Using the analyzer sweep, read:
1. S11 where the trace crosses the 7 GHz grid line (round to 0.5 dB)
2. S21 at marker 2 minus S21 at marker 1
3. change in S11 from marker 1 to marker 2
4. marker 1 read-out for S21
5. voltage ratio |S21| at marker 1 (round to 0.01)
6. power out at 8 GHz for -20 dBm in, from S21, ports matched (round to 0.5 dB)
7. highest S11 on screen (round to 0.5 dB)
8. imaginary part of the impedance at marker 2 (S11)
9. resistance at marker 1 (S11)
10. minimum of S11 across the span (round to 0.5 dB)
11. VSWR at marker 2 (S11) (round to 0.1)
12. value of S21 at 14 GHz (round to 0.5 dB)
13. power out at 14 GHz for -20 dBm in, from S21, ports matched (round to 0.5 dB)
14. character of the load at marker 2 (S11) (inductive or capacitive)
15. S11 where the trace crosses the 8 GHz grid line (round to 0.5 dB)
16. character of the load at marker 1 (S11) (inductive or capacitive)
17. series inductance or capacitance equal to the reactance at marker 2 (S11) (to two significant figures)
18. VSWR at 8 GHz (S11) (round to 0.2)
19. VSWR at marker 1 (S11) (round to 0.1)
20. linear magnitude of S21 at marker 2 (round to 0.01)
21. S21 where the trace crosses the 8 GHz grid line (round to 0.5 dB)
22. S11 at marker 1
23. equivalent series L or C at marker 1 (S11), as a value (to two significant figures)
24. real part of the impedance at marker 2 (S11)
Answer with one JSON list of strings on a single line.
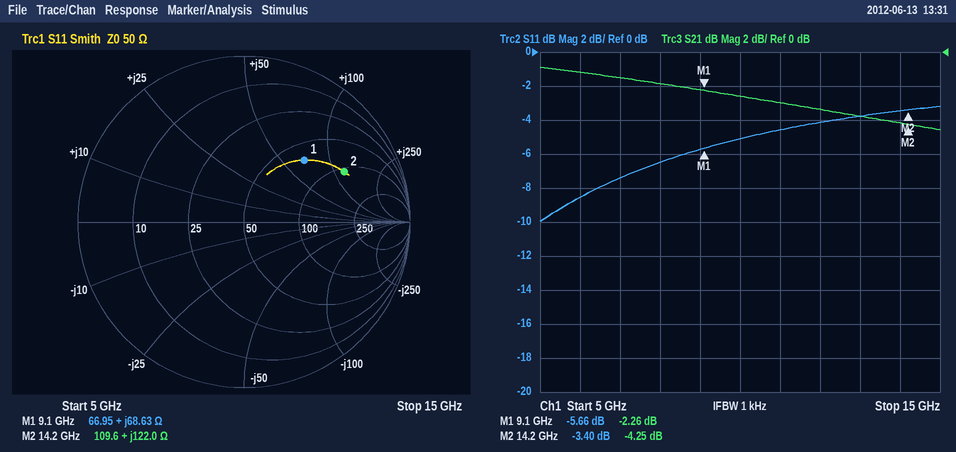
["-7.5 dB", "-1.99 dB", "2.26 dB", "-2.26 dB", "0.77", "-22.0 dBm", "-3.0 dB", "+122.0 Ω", "66.95 Ω", "-10.0 dB", "5.2", "-4.0 dB", "-24.0 dBm", "inductive", "-6.5 dB", "inductive", "1.4 nH", "2.8", "3.2", "0.61", "-2.0 dB", "-5.66 dB", "1.2 nH", "109.6 Ω"]
